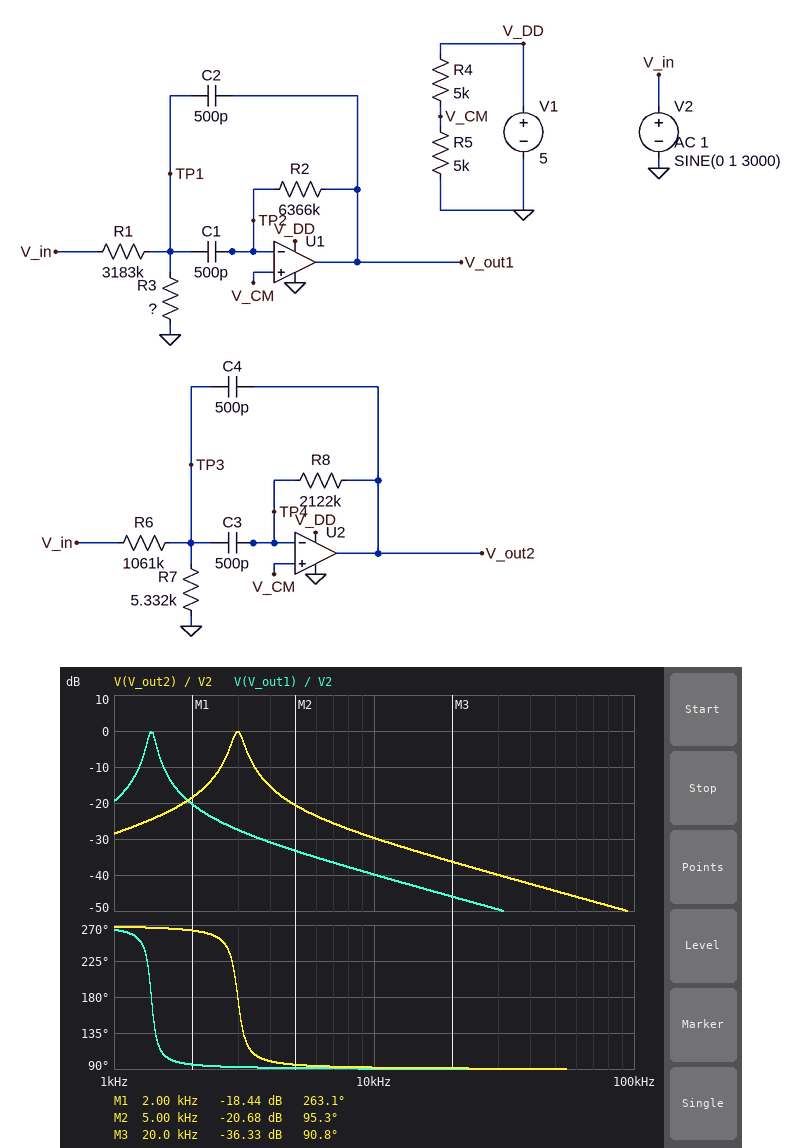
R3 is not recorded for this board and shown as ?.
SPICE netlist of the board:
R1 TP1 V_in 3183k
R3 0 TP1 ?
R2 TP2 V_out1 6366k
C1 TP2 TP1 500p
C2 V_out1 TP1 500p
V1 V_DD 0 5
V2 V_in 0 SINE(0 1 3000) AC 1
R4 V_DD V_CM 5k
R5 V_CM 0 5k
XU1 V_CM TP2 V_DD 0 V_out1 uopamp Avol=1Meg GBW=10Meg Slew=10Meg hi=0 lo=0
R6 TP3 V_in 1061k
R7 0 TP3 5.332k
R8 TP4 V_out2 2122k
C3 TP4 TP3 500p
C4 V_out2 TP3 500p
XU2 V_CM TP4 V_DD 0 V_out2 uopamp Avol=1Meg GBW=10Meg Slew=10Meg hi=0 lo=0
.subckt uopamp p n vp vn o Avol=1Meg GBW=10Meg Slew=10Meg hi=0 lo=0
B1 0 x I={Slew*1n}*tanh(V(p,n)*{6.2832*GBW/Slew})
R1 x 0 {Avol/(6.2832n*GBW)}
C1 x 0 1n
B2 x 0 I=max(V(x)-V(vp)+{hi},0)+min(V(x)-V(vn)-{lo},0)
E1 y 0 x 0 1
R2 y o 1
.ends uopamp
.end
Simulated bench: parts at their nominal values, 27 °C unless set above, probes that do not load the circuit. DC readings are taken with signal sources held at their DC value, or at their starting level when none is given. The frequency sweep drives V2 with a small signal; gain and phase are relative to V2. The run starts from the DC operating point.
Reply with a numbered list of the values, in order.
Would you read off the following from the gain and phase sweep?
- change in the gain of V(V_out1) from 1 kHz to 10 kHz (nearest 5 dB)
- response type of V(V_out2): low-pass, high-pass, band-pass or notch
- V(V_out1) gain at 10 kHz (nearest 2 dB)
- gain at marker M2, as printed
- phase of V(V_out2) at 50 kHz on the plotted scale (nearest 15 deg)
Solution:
1. -20 dB
2. band-pass
3. -40 dB
4. -20.68 dB
5. 90 deg
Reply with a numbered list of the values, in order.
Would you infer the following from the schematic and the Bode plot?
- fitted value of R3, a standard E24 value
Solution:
1. 8.2 kΩ
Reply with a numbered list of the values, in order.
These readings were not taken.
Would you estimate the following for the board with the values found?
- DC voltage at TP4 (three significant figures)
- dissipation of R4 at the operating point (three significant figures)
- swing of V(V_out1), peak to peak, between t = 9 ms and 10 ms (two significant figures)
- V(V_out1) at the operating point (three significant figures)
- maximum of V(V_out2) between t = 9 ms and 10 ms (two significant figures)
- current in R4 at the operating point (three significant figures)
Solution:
1. 2.50 V
2. 1.25 mW
3. 87 mV
4. 2.50 V
5. 3.5 V
6. 500 µA
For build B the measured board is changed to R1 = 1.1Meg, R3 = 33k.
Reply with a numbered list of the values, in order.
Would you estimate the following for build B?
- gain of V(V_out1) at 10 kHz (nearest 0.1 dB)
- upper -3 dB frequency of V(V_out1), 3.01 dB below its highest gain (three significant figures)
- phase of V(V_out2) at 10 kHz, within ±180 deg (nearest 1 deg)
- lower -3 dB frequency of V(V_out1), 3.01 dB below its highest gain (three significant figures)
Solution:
1. -30.7 dB
2. 756 Hz
3. 92 deg
4. 656 Hz
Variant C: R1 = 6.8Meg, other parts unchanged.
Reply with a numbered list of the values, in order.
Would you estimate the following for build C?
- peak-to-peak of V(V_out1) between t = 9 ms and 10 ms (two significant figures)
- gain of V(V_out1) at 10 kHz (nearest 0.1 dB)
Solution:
1. 41 mV
2. -46.5 dB
